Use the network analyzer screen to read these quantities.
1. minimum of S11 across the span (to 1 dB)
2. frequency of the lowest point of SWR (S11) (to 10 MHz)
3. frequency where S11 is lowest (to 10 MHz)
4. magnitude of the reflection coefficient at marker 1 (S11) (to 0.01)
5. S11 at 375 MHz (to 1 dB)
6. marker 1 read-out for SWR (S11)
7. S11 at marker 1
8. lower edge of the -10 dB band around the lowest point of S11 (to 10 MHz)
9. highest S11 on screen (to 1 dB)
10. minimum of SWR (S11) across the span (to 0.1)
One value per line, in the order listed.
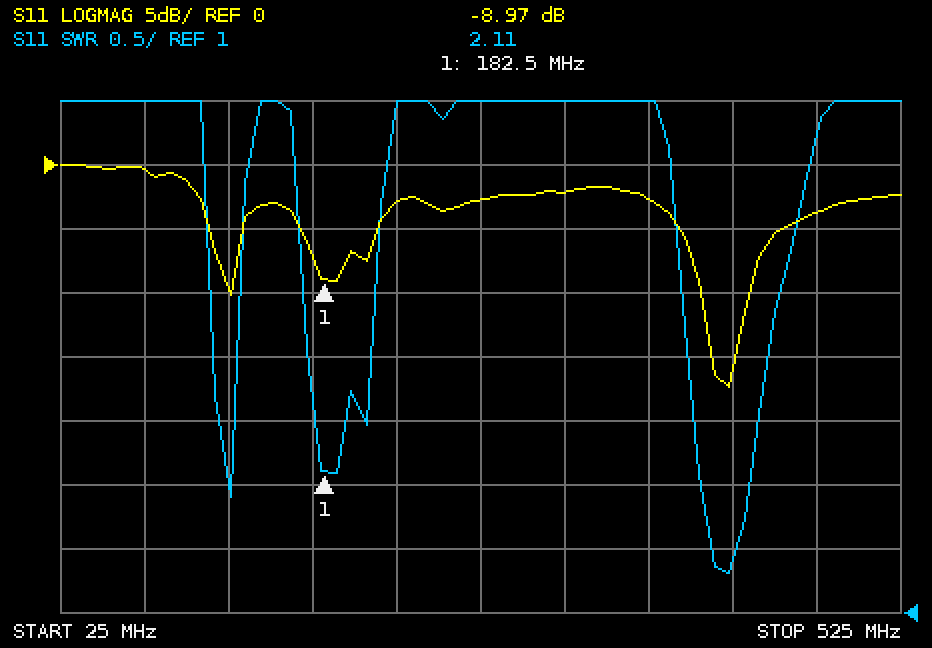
-17 dB
420 MHz
420 MHz
0.36
-3 dB
2.11
-8.97 dB
410 MHz
0 dB
1.3
